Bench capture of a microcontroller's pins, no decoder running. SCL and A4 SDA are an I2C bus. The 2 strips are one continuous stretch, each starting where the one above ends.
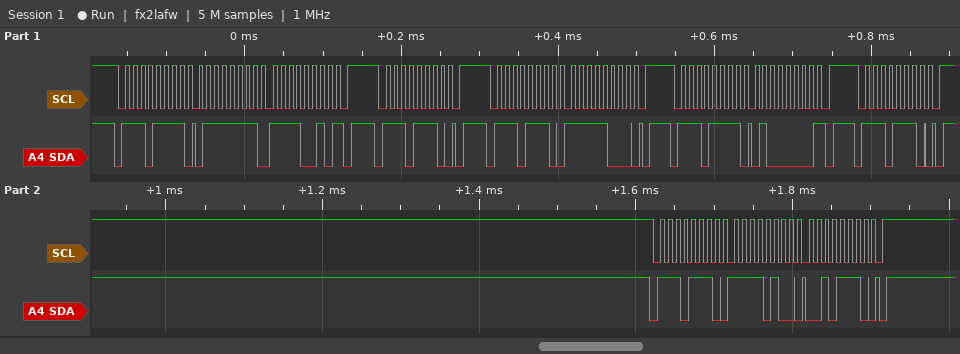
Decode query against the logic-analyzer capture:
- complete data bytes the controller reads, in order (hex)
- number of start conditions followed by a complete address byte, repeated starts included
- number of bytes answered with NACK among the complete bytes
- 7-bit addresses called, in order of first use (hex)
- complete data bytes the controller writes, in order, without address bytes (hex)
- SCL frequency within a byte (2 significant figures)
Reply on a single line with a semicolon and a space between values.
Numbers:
7F F2 40; 6; 2; 0x77; F8 F4 2E; 100 kHz
